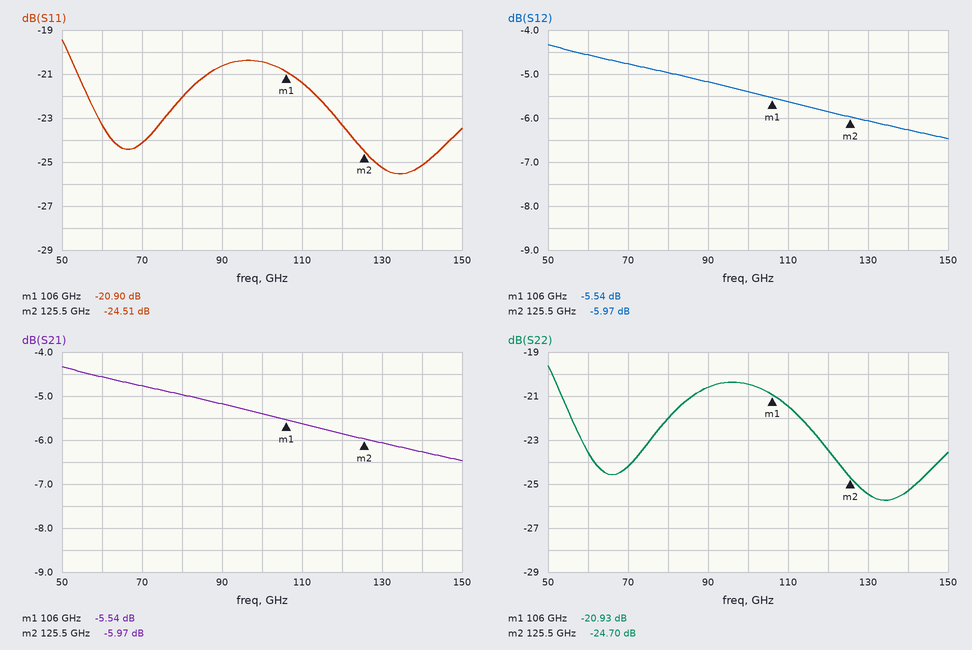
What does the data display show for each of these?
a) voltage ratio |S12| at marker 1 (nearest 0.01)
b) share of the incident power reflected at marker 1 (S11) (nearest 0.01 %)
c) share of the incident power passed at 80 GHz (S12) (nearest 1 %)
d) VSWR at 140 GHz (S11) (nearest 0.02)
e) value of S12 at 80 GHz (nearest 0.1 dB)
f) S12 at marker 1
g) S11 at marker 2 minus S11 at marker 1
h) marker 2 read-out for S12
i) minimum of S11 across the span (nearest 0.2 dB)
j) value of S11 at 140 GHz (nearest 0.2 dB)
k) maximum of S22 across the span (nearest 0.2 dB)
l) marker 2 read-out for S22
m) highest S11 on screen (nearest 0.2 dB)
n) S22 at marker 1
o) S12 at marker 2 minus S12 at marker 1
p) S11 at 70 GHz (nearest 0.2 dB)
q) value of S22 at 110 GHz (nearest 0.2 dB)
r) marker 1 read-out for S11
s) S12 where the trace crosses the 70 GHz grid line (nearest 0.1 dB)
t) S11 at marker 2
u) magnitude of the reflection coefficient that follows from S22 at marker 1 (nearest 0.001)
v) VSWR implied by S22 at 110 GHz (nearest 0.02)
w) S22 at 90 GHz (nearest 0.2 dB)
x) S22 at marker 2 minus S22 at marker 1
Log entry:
0.53
0.81 %
32 %
1.12
-5.0 dB
-5.54 dB
-3.61 dB
-5.97 dB
-25.6 dB
-25.2 dB
-19.6 dB
-24.70 dB
-19.4 dB
-20.93 dB
-0.43 dB
-24.2 dB
-21.4 dB
-20.90 dB
-4.8 dB
-24.51 dB
0.090
1.18
-20.6 dB
-3.77 dB
